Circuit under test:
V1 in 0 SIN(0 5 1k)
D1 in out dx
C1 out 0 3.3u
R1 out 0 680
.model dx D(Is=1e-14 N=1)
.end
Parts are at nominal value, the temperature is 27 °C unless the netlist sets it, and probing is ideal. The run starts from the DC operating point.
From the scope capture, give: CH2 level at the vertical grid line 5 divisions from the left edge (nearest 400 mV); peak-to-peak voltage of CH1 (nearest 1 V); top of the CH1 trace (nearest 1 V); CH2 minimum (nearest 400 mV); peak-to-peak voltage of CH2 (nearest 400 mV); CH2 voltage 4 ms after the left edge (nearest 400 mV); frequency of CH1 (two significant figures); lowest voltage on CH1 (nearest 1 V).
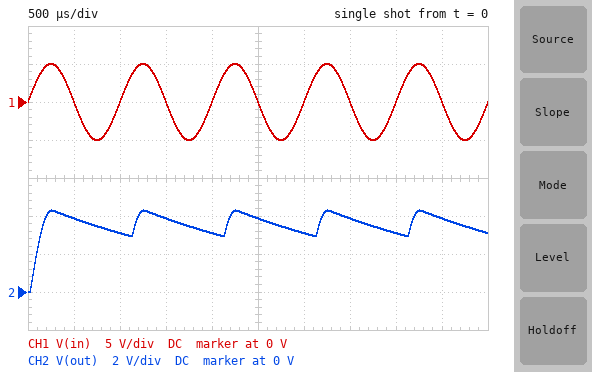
4.0 V
10 V
5 V
0 V
4.4 V
3.2 V
1.0 kHz
-5 V
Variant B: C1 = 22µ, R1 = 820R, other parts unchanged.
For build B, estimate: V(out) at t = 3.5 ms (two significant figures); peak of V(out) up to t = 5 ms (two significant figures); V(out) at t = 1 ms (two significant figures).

4.2 V
4.3 V
4.1 V
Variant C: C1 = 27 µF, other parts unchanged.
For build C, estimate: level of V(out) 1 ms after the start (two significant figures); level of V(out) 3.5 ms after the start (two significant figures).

4.1 V
4.2 V
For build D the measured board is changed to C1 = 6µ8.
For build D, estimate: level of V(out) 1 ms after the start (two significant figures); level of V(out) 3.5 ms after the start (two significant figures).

3.7 V
4.1 V
